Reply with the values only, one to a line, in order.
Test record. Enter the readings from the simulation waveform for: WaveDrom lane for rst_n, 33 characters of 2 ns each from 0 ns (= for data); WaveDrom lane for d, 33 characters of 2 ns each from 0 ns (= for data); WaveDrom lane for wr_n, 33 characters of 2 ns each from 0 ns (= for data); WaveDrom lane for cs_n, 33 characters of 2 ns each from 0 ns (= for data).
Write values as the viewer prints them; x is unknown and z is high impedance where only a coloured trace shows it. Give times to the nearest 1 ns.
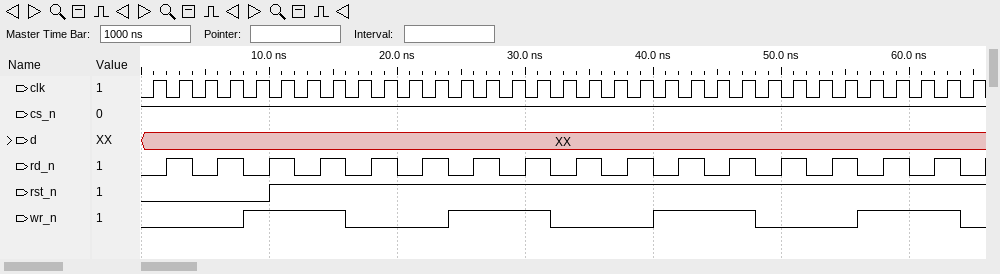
{name: 'rst_n', wave: '0....1...........................'}
{name: 'd', wave: 'x................................'}
{name: 'wr_n', wave: '0...1...0...1...0...1...0...1...0'}
{name: 'cs_n', wave: '1................................'}
